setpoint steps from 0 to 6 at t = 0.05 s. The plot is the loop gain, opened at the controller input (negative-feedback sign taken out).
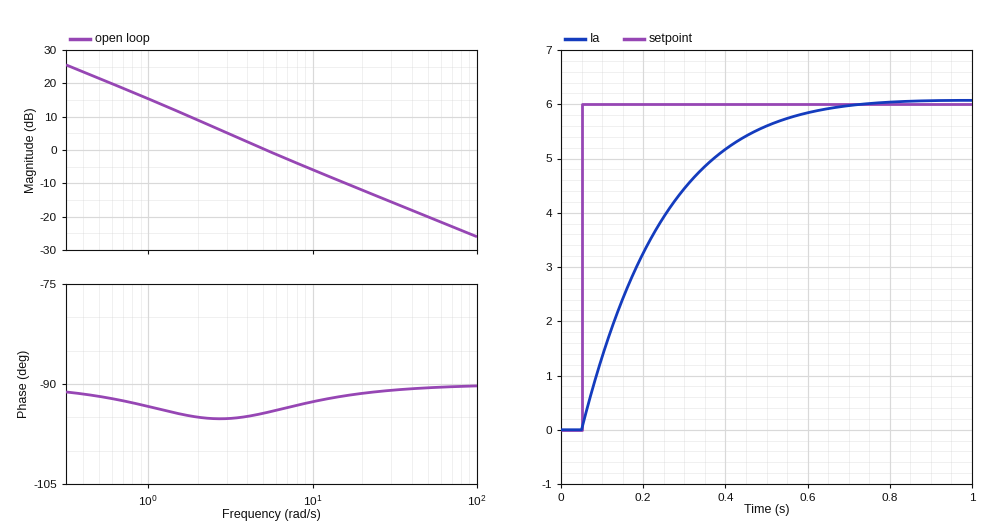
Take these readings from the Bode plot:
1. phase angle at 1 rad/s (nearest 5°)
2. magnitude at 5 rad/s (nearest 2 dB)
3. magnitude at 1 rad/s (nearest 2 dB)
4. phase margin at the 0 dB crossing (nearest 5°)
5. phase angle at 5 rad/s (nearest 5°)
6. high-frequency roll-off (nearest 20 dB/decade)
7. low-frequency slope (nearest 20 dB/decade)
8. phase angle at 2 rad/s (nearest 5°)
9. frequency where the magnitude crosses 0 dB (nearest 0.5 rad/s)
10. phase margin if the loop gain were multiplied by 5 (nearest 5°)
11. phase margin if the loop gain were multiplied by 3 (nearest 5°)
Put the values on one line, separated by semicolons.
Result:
-95°; 0 dB; 16 dB; 85°; -95°; -20 dB/decade; -20 dB/decade; -95°; 5.0 rad/s; 90°; 90°
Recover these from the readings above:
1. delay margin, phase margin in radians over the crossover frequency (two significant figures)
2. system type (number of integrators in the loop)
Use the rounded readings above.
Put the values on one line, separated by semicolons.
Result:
0.30 s; 1
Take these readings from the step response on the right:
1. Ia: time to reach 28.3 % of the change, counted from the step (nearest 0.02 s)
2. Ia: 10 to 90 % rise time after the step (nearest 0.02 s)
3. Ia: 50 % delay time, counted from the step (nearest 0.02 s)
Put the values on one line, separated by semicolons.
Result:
0.06 s; 0.38 s; 0.14 s
